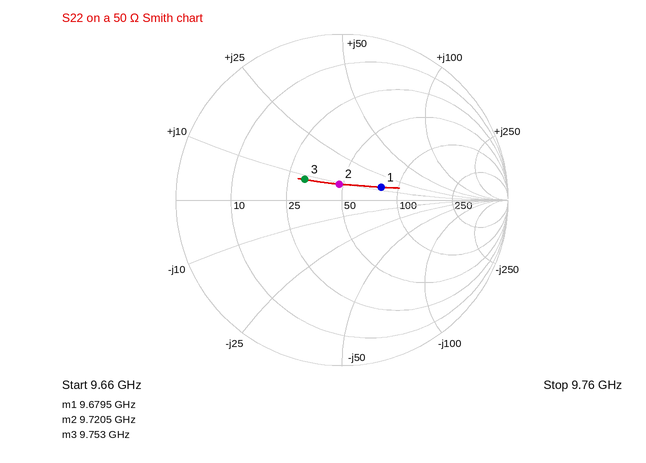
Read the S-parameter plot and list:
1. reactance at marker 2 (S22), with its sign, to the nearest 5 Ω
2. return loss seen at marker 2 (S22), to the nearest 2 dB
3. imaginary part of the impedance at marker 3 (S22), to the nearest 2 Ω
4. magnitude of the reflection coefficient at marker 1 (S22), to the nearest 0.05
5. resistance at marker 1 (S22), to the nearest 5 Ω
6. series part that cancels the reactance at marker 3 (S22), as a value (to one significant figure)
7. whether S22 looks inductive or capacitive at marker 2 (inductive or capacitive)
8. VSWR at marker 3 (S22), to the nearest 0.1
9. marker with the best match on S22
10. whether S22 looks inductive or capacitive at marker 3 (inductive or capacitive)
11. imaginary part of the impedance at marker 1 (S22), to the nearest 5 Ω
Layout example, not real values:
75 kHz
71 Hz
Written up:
+10 Ω
20 dB
+8 Ω
0.25
80 Ω
2 pF
inductive
1.7
marker 2
inductive
+15 Ω
